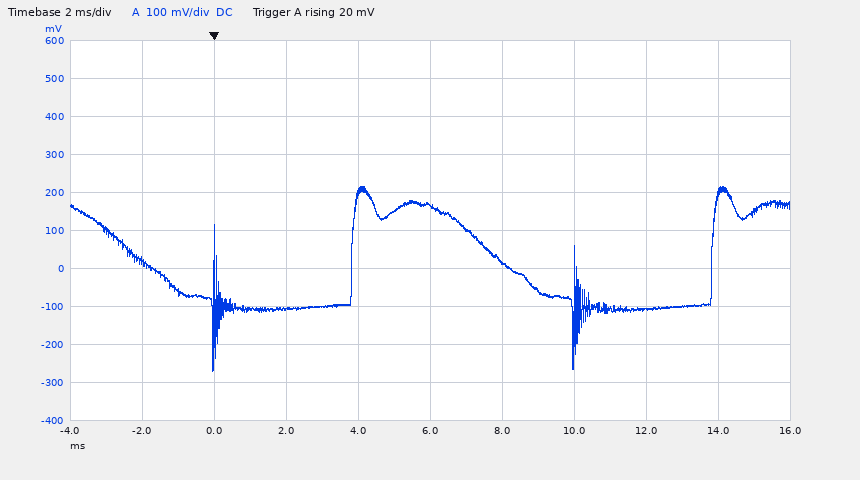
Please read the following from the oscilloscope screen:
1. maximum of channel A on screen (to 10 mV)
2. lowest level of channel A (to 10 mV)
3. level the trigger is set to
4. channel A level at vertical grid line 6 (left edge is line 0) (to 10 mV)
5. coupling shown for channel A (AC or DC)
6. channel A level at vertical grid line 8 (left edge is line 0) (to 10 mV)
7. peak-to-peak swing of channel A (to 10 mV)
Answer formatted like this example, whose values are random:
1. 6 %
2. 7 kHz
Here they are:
1. 220 mV
2. -270 mV
3. 20 mV
4. 20 mV
5. DC
6. -110 mV
7. 490 mV
